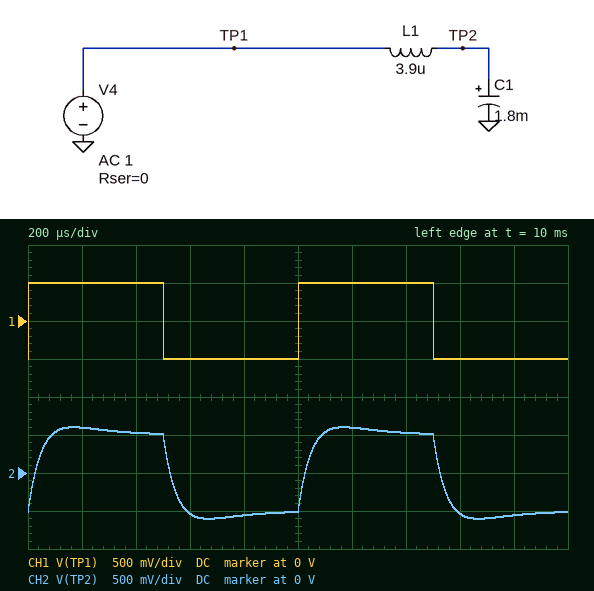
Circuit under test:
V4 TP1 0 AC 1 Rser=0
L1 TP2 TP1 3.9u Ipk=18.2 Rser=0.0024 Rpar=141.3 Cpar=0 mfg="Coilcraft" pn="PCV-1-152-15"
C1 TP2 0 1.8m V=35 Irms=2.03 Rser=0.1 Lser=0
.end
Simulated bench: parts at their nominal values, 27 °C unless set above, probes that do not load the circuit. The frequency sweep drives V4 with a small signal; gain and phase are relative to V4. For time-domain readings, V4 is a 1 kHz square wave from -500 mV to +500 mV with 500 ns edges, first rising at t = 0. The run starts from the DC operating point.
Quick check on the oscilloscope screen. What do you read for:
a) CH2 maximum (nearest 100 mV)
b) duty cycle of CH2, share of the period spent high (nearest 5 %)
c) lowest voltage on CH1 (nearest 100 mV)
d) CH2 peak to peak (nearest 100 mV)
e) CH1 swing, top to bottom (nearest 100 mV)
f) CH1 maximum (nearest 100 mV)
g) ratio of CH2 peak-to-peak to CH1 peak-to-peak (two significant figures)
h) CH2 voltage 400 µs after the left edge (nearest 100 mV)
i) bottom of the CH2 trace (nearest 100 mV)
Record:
600 mV
50 %
-500 mV
1.2 V
1.0 V
500 mV
1.2
500 mV
-600 mV
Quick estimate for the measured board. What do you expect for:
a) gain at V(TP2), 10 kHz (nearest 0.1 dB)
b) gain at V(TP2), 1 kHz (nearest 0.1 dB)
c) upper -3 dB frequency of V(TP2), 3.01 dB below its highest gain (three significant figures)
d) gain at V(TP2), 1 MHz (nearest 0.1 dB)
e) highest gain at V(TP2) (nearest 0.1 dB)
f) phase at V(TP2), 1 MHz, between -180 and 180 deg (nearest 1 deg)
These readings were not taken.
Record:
-8.2 dB
0.9 dB
4.13 kHz
-47.7 dB
0.9 dB
-80 deg
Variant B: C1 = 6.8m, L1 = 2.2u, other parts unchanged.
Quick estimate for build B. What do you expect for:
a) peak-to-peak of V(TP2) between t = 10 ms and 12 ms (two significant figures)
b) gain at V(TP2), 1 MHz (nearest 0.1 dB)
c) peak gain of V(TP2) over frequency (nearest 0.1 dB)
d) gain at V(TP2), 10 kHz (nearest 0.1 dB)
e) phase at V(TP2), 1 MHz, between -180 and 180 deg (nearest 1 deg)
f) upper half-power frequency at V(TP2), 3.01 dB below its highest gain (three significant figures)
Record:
1.0 V
-42.8 dB
0 dB
-4.6 dB
-84 deg
7.22 kHz
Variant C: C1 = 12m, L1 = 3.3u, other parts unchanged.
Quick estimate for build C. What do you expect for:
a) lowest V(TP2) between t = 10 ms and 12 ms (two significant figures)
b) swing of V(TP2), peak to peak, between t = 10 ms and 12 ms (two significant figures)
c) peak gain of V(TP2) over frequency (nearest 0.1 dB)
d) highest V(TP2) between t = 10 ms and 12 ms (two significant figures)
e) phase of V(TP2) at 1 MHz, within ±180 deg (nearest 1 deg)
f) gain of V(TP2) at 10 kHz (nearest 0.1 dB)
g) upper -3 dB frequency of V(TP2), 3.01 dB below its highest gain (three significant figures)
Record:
-500 mV
1.0 V
0 dB
500 mV
-81 deg
-7.2 dB
4.82 kHz
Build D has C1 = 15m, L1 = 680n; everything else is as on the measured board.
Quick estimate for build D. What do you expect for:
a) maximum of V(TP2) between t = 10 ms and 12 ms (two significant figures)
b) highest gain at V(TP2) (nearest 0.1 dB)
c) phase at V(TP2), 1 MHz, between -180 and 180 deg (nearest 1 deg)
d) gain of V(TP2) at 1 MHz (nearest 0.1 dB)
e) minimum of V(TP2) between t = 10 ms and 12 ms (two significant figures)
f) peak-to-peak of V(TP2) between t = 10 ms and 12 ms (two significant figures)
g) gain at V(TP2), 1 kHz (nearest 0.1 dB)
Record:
490 mV
0 dB
-87 deg
-32.6 dB
-490 mV
980 mV
-0.2 dB
